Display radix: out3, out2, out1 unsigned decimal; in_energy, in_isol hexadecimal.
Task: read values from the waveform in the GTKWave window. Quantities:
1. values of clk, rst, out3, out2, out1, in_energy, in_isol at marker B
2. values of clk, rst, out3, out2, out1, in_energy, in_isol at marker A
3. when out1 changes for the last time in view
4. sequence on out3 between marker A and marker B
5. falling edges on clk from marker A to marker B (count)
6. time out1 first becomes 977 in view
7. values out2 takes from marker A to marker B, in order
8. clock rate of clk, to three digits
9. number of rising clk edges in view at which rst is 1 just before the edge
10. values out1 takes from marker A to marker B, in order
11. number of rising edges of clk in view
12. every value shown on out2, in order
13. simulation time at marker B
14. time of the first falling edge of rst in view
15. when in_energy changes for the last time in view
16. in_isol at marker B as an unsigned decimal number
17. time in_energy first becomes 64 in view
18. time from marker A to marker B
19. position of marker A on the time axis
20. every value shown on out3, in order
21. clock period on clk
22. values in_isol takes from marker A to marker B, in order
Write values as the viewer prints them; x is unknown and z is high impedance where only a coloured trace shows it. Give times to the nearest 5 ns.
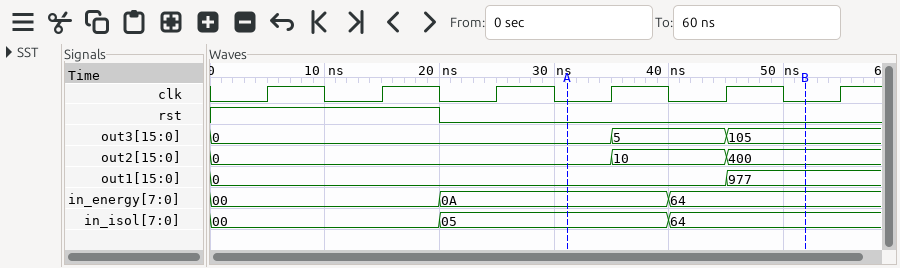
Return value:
clk=0, rst=0, out3=105, out2=400, out1=977, in_energy=64, in_isol=64
clk=0, rst=0, out3=0, out2=0, out1=0, in_energy=0A, in_isol=05
45 ns
0, 5, 105
2
45 ns
0, 10, 400
100 MHz
2
0, 977
6
0, 10, 400
50 ns
20 ns
40 ns
100
40 ns
20 ns
30 ns
0, 5, 105
10 ns
05, 64
